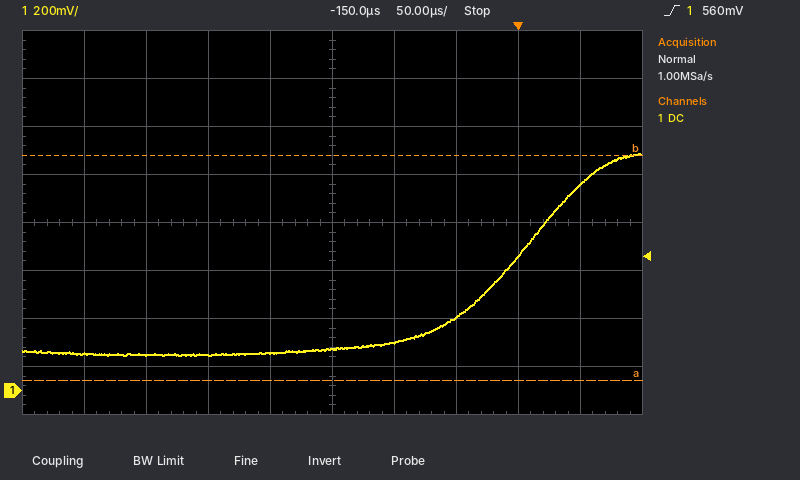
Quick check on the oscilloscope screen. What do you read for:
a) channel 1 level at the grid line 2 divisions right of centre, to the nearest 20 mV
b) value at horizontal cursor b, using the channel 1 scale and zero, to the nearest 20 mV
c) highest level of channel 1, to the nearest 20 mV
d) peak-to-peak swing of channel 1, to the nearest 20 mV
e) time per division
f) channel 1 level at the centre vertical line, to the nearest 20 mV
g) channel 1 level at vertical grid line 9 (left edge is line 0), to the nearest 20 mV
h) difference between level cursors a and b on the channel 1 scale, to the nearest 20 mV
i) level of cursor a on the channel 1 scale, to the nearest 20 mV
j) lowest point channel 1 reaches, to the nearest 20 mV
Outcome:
300 mV
980 mV
980 mV
840 mV
50 µs
180 mV
860 mV
940 mV
40 mV
140 mV
